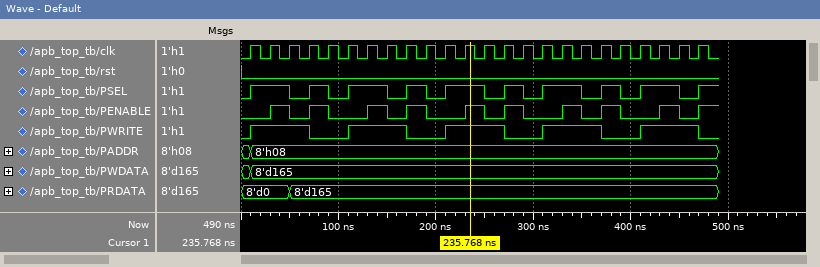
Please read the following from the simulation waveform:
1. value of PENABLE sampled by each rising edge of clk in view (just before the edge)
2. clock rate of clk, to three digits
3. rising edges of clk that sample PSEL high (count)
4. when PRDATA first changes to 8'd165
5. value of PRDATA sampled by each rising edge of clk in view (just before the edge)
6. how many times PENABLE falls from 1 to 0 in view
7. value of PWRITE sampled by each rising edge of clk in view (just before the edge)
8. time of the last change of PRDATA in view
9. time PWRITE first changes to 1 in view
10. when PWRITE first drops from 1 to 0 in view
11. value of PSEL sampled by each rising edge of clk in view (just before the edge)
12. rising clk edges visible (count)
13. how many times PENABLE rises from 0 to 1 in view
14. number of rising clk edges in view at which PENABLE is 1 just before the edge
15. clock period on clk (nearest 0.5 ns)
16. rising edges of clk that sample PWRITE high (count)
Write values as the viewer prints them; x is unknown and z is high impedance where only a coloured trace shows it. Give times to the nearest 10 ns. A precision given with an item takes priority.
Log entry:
0 0 1 0 1 0 0 1 0 1 0 0 1 0 1 0 0 1 0 1 0 0 1 0
50.0 MHz
14
50 ns
8'd0, 8'd0, 8'd0, 8'd165, 8'd165, 8'd165, 8'd165, 8'd165, 8'd165, 8'd165, 8'd165, 8'd165, 8'd165, 8'd165, 8'd165, 8'd165, 8'd165, 8'd165, 8'd165, 8'd165, 8'd165, 8'd165, 8'd165, 8'd165
9
0 1 1 1 0 0 1 1 1 0 0 1 1 1 0 0 1 1 1 0 0 1 1 1
50 ns
10 ns
70 ns
0 1 1 0 1 0 1 1 0 1 0 1 1 0 1 0 1 1 0 1 0 1 1 0
24
10
9
20 ns
15
